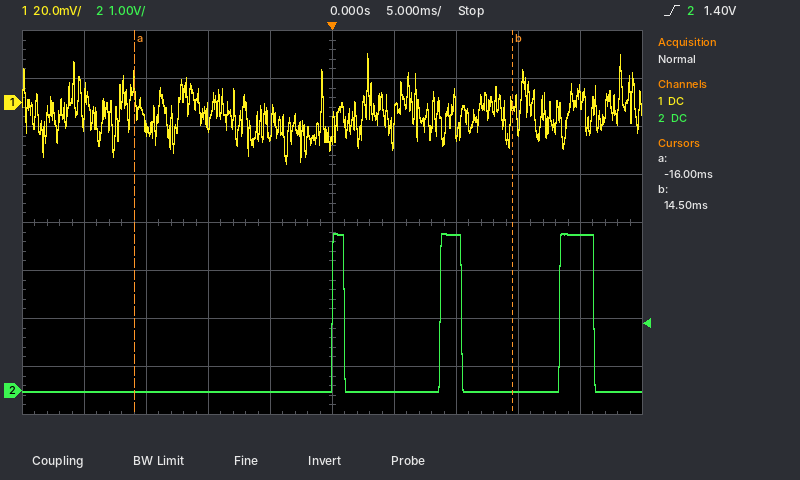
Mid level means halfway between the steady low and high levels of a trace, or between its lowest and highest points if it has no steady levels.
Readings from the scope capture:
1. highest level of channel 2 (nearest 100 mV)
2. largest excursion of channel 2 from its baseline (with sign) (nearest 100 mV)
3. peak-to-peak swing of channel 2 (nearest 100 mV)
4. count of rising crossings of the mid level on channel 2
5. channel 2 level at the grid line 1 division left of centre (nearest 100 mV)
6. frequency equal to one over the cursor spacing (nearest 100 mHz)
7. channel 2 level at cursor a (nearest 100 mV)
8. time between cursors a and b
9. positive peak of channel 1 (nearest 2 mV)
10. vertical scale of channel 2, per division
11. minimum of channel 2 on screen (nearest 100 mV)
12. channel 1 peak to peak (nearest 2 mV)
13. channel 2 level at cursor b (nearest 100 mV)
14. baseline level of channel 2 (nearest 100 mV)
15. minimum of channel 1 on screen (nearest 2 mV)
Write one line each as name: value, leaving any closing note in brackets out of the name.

highest level of channel 2: 3.3 V
largest excursion of channel 2 from its baseline (with sign): +3.3 V
peak-to-peak swing of channel 2: 3.3 V
count of rising crossings of the mid level on channel 2: 3
channel 2 level at the grid line 1 division left of centre: 0.0 V
frequency equal to one over the cursor spacing: 32.8 Hz
channel 2 level at cursor a: 0.0 V
time between cursors a and b: 30.5 ms
positive peak of channel 1: 20 mV
vertical scale of channel 2, per division: 1 V
minimum of channel 2 on screen: 0.0 V
channel 1 peak to peak: 46 mV
channel 2 level at cursor b: 0.0 V
baseline level of channel 2: 0.0 V
minimum of channel 1 on screen: -26 mV
